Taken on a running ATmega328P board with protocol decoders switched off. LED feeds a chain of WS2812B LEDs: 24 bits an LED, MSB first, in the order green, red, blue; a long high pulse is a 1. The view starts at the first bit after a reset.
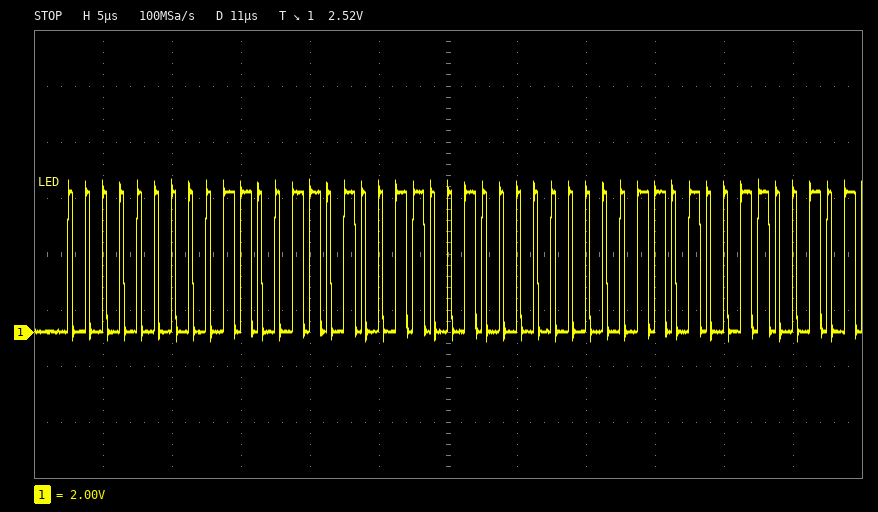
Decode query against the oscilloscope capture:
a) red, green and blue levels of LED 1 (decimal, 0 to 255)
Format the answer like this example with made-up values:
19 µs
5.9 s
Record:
102, 0, 153
